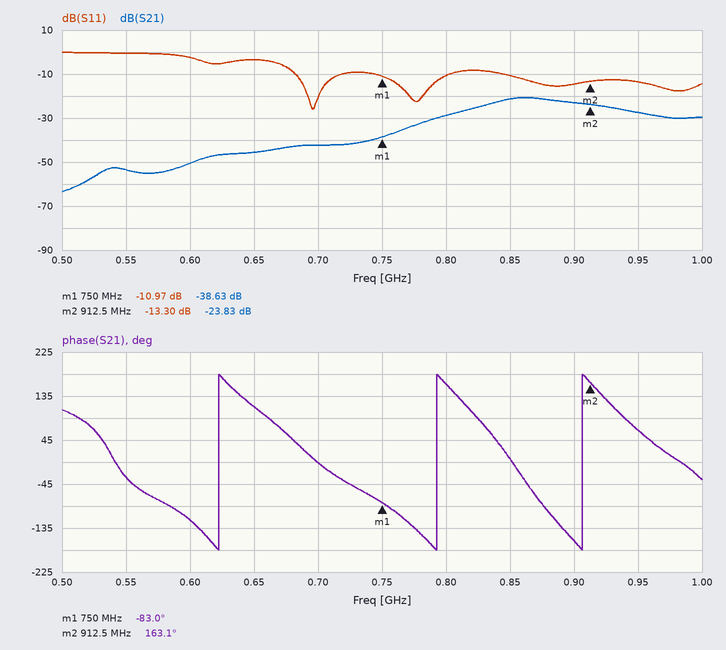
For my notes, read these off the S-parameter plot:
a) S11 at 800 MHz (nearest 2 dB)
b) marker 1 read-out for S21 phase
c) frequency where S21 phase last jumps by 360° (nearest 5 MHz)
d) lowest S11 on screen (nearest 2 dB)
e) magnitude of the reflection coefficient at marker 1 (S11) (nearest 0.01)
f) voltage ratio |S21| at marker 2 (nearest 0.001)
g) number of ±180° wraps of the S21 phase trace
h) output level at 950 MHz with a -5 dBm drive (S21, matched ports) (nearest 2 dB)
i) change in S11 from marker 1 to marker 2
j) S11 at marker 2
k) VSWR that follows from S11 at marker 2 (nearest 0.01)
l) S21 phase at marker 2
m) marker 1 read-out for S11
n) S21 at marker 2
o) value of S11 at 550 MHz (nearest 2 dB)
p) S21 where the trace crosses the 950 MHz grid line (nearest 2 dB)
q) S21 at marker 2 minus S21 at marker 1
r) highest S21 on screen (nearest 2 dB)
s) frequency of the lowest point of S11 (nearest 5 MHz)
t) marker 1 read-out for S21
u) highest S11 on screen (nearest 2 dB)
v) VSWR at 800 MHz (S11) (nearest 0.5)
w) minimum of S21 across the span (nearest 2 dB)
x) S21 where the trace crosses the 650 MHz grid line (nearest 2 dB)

-10 dB
-83.0°
905 MHz
-26 dB
0.28
0.064
3
-32 dBm
-2.33 dB
-13.30 dB
1.55
163.1°
-10.97 dB
-23.83 dB
0 dB
-28 dB
14.80 dB
-20 dB
695 MHz
-38.63 dB
0 dB
2.0
-64 dB
-46 dB
